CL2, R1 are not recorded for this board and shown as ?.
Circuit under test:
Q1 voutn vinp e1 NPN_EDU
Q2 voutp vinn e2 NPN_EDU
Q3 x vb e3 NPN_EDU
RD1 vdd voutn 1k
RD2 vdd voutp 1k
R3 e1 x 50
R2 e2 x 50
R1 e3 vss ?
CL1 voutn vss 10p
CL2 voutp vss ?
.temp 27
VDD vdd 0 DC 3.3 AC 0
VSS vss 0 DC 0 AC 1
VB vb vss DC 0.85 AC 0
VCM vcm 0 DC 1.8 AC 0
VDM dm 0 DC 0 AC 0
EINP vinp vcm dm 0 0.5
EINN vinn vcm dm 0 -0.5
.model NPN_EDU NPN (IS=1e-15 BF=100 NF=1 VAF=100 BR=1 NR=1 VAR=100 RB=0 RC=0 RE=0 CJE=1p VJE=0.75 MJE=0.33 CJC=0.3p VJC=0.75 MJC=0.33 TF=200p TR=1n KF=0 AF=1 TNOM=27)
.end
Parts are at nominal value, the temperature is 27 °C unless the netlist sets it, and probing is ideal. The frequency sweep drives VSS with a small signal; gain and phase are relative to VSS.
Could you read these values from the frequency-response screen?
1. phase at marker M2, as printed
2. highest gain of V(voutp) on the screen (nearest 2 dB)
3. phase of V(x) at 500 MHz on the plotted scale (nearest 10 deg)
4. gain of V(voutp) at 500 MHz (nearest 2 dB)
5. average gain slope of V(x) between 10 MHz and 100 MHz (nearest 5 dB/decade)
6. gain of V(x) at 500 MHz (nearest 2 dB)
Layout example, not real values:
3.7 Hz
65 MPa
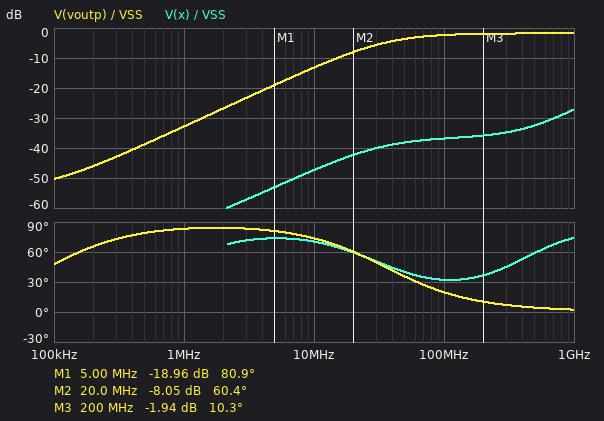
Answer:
60.4 deg
-2 dB
60 deg
-2 dB
10 dB/decade
-32 dB
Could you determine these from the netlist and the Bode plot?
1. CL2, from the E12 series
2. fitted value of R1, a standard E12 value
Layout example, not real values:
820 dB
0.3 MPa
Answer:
8.2 pF
22 Ω
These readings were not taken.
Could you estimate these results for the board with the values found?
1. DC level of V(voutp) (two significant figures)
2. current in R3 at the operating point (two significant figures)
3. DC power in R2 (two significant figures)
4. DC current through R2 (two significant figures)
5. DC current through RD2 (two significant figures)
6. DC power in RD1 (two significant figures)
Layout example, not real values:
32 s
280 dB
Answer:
1.2 V
2.2 mA
240 µW
2.2 mA
2.1 mA
4.5 mW
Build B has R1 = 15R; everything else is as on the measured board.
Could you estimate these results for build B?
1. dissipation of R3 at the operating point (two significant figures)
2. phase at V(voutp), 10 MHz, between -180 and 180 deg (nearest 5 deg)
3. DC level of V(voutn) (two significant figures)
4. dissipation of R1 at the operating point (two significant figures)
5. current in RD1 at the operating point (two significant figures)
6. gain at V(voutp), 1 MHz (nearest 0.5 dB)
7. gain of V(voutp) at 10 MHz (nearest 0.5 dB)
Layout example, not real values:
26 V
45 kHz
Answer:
430 µW
85 deg
1.1 V
530 µW
2.2 mA
-54.5 dB
-34.5 dB
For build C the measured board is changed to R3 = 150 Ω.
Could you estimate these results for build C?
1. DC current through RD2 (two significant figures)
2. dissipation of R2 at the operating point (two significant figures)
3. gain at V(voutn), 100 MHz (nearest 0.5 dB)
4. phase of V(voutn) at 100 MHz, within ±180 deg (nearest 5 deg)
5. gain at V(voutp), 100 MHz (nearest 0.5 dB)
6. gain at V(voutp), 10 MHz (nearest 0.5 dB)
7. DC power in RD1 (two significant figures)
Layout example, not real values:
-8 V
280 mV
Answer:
2.2 mA
490 µW
0 dB
10 deg
-19.0 dB
-36.5 dB
1.5 mW
